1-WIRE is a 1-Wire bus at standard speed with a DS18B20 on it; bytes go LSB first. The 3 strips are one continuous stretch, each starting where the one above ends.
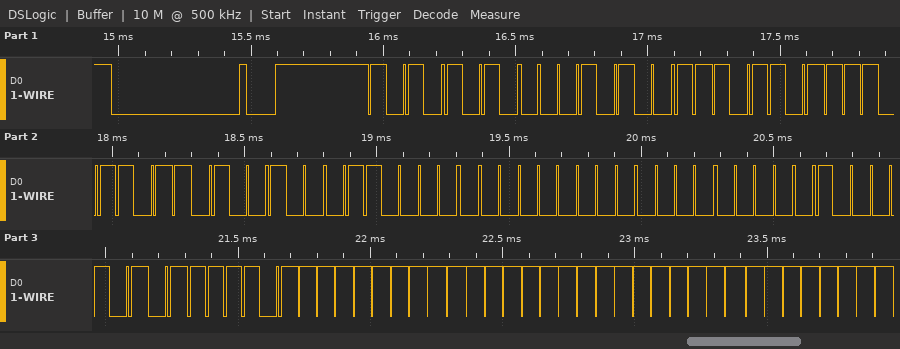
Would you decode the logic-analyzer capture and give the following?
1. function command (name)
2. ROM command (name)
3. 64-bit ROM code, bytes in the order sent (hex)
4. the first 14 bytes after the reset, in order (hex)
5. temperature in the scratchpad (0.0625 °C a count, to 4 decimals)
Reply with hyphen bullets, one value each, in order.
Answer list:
- Read Scratchpad
- Match ROM
- 28 B7 B7 25 06 00 00 A2
- 55 28 B7 B7 25 06 00 00 A2 BE FF FF FF FF
- -0.0625 °C
